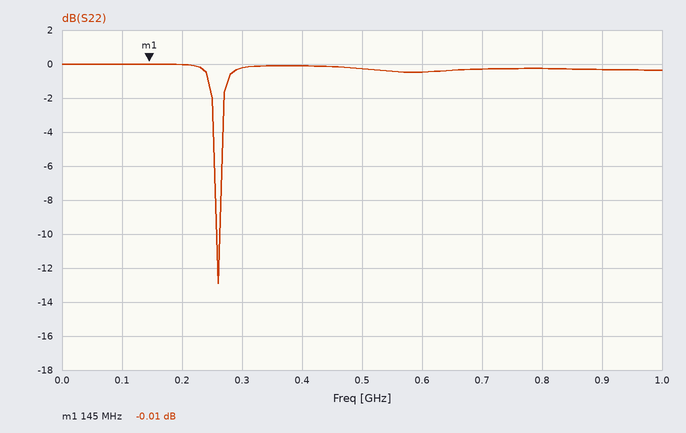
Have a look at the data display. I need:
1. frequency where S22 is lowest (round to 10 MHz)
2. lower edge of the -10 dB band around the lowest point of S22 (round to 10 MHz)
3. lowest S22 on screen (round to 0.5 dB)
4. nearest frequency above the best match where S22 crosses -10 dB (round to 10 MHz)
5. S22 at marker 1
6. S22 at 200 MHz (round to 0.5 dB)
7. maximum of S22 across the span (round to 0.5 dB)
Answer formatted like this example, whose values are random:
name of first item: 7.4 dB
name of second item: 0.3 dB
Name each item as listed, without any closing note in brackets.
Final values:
frequency where S22 is lowest: 260 MHz
lower edge of the -10 dB band around the lowest point of S22: 260 MHz
lowest S22 on screen: -13.0 dB
nearest frequency above the best match where S22 crosses -10 dB: 260 MHz
S22 at marker 1: -0.01 dB
S22 at 200 MHz: 0.0 dB
maximum of S22 across the span: 0.0 dB
